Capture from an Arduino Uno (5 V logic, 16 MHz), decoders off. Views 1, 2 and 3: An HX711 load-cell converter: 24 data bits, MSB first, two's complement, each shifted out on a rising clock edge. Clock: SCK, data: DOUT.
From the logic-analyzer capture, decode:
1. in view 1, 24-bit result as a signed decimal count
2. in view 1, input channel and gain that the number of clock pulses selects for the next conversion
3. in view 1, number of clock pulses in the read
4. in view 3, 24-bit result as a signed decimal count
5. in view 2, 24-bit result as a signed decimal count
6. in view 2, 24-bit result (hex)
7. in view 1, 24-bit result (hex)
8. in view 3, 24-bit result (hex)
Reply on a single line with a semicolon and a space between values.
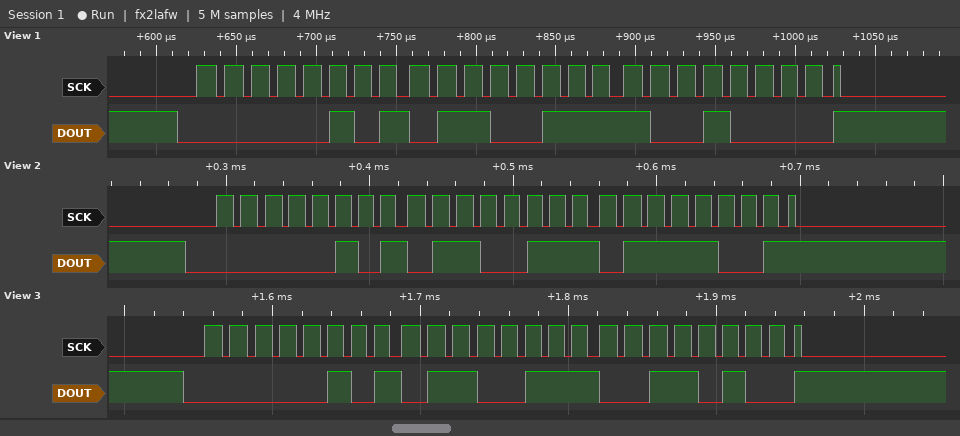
354192; channel A, gain 128; 25; 354100; 354169; 0x056779; 0x056790; 0x056734
